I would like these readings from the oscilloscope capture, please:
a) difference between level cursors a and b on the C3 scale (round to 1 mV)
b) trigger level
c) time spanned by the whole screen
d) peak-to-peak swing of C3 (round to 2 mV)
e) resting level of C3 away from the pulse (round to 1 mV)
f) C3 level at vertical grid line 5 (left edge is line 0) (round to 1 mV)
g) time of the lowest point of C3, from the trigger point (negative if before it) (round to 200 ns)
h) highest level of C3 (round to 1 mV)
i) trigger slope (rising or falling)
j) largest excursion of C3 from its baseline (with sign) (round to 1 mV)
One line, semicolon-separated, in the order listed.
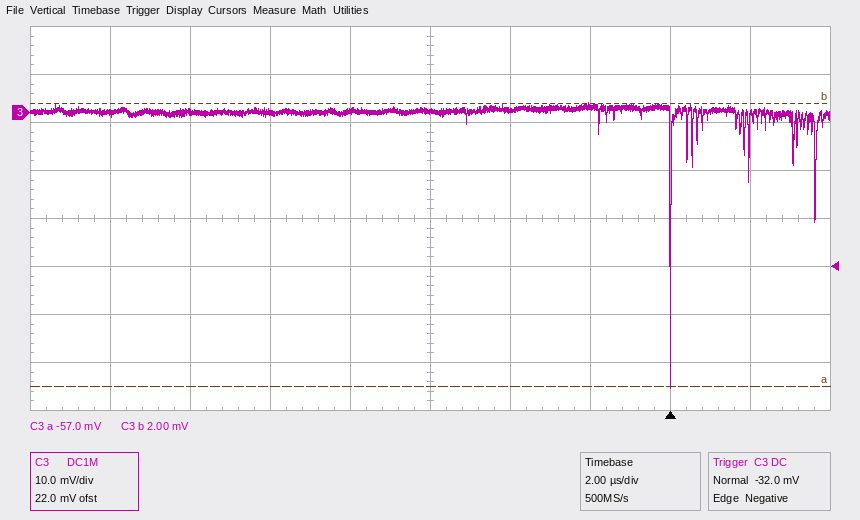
59 mV; -32.0 mV; 20 µs; 60 mV; 0 mV; 0 mV; 0.0 µs; 2 mV; falling; -58 mV
